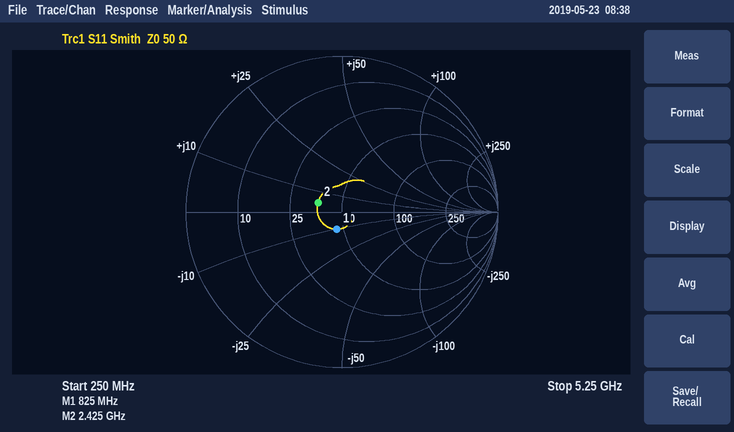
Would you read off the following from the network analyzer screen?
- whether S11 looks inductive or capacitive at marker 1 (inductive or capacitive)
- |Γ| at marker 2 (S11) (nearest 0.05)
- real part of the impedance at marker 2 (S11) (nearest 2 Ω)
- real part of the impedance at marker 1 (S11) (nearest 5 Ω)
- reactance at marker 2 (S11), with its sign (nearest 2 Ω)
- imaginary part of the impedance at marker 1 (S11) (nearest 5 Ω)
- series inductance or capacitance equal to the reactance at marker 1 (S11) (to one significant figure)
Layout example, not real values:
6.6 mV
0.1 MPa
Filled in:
capacitive
0.15
36 Ω
45 Ω
+4 Ω
-10 Ω
20 pF
